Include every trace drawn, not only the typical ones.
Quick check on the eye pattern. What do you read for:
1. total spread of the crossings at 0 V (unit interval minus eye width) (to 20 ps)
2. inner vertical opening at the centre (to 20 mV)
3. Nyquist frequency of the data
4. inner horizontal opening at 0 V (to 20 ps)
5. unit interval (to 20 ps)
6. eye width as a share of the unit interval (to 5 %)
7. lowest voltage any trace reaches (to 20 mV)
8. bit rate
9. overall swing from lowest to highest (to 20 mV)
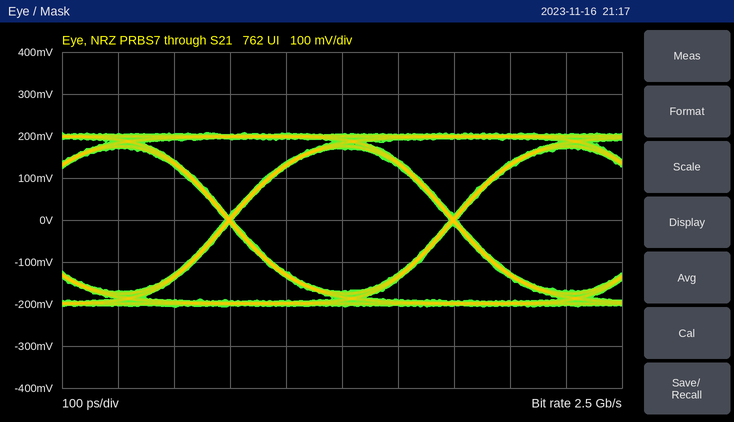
20 ps
340 mV
1.25 GHz
380 ps
400 ps
95 %
-200 mV
2.5 Gb/s
420 mV
